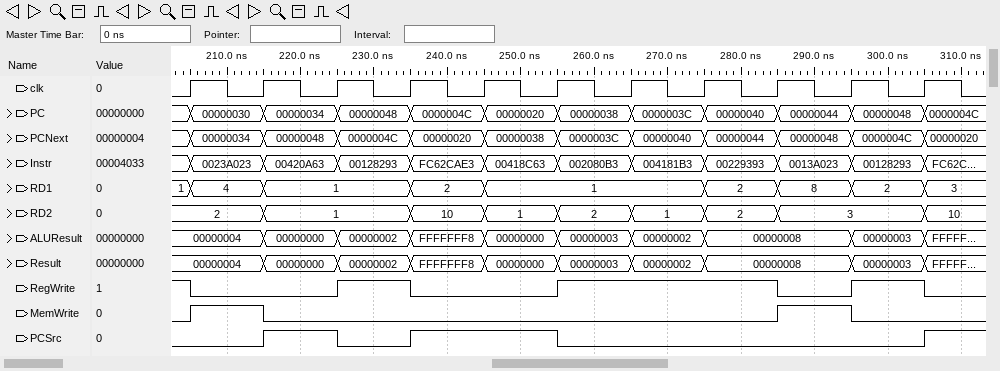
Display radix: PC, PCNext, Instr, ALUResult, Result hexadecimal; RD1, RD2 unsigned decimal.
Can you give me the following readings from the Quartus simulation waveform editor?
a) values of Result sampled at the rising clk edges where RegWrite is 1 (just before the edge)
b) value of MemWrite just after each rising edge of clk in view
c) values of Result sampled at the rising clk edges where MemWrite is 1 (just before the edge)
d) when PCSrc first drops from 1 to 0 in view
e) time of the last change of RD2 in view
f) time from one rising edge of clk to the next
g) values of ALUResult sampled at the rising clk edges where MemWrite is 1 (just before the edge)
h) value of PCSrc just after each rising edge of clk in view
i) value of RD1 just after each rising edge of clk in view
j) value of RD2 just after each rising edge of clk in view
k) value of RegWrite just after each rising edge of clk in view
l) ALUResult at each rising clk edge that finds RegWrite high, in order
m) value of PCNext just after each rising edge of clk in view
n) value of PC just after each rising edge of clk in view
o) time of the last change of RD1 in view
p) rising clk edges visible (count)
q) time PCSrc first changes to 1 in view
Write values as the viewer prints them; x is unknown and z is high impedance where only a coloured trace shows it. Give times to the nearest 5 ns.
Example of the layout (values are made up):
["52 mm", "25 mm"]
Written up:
["00000004, 00000002, 00000003, 00000002, 00000008, 00000003", "1 0 0 0 0 0 0 0 1 0 0", "00000004, 00000008", "225 ns", "305 ns", "10 ns", "00000004, 00000008", "0 1 0 1 1 0 0 0 0 0 1", "4, 1, 1, 2, 1, 1, 1, 2, 8, 2, 3", "2, 1, 1, 10, 1, 2, 1, 2, 3, 3, 10", "0 0 1 0 0 1 1 1 0 1 0", "00000004, 00000002, 00000003, 00000002, 00000008, 00000003", "00000034, 00000048, 0000004C, 00000020, 00000038, 0000003C, 00000040, 00000044, 00000048, 0000004C, 00000020", "00000030, 00000034, 00000048, 0000004C, 00000020, 00000038, 0000003C, 00000040, 00000044, 00000048, 0000004C", "305 ns", "11", "215 ns"]
